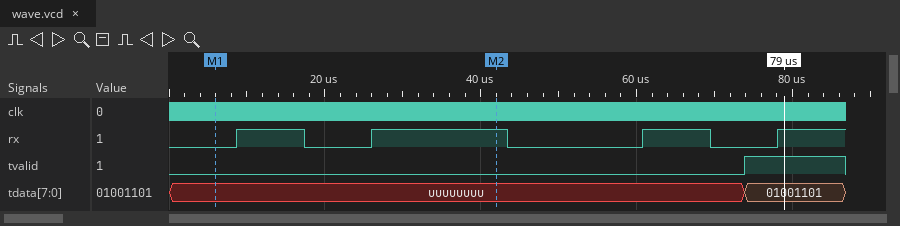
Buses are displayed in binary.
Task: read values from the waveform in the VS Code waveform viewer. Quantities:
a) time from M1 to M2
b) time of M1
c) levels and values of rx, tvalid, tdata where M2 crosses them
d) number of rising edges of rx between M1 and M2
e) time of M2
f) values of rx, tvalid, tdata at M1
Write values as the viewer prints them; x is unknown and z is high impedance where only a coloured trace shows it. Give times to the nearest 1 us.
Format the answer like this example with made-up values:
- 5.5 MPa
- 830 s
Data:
- 36 us
- 6 us
- rx=1, tvalid=0, tdata=uuuuuuuu
- 2
- 42 us
- rx=0, tvalid=0, tdata=uuuuuuuu
